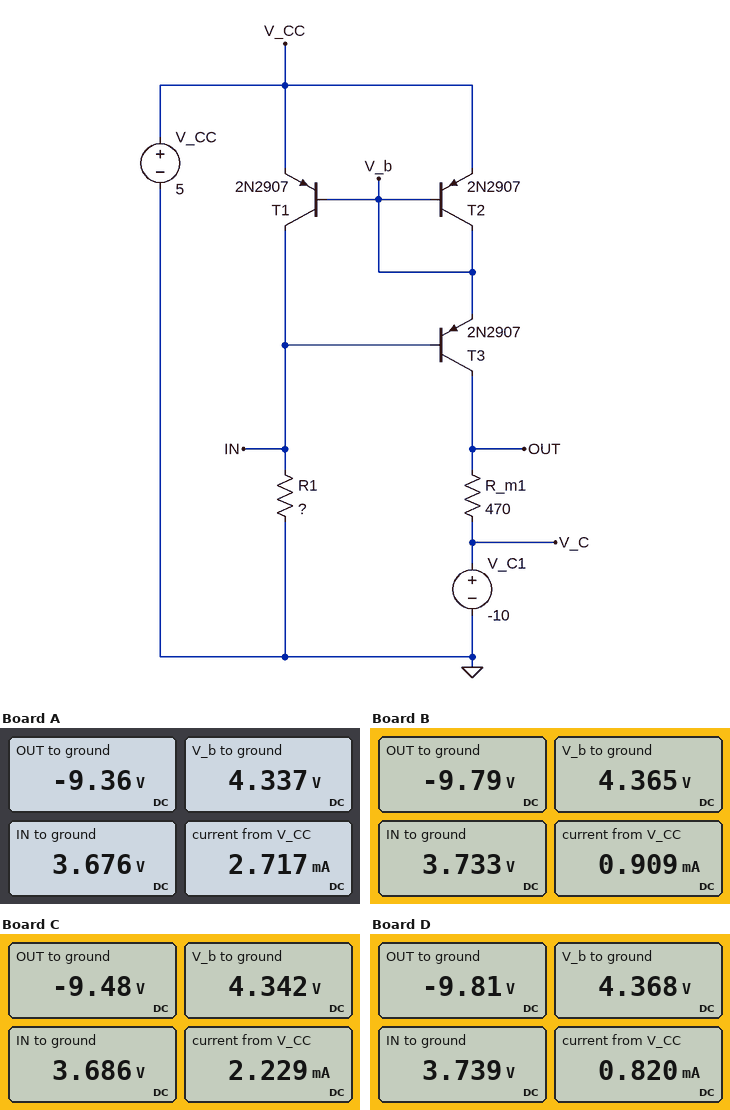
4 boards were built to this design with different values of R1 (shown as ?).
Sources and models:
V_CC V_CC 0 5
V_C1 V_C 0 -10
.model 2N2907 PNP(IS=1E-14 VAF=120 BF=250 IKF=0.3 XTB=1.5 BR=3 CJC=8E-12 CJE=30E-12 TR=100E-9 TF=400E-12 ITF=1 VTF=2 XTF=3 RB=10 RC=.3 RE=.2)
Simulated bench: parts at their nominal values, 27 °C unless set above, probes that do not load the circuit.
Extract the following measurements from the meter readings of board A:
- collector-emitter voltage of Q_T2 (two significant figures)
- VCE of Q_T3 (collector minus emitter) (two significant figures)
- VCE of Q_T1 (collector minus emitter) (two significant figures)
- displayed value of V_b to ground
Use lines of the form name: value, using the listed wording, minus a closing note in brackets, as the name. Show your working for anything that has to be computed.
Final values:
collector-emitter voltage of Q_T2: 4.337 V - 5 V = -660 mV
VCE of Q_T3 (collector minus emitter): -9.36 V - 4.337 V = -14 V
VCE of Q_T1 (collector minus emitter): 3.676 V - 5 V = -1.3 V
displayed value of V_b to ground: 4.337 V
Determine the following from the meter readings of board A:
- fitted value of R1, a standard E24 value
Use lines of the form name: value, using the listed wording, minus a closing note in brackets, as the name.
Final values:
fitted value of R1, a standard E24 value: 2.7 kΩ
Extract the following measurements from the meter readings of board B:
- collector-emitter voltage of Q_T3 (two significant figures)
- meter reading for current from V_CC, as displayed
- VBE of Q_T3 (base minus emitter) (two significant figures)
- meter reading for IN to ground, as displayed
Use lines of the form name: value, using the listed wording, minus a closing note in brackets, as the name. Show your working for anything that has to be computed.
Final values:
collector-emitter voltage of Q_T3: -9.79 V - 4.365 V = -14 V
meter reading for current from V_CC, as displayed: 0.909 mA
VBE of Q_T3 (base minus emitter): 3.733 V - 4.365 V = -630 mV
meter reading for IN to ground, as displayed: 3.733 V
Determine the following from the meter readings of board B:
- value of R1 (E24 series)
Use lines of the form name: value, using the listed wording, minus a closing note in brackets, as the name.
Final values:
value of R1: 8.2 kΩ
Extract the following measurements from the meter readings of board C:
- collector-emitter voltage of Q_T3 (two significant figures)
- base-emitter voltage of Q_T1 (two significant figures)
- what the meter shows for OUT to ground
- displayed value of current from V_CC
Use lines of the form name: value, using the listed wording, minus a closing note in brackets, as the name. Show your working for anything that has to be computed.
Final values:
collector-emitter voltage of Q_T3: -9.48 V - 4.342 V = -14 V
base-emitter voltage of Q_T1: 4.342 V - 5 V = -660 mV
what the meter shows for OUT to ground: -9.48 V
displayed value of current from V_CC: 2.229 mA
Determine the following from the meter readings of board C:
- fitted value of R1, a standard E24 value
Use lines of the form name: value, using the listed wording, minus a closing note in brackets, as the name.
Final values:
fitted value of R1, a standard E24 value: 3.3 kΩ
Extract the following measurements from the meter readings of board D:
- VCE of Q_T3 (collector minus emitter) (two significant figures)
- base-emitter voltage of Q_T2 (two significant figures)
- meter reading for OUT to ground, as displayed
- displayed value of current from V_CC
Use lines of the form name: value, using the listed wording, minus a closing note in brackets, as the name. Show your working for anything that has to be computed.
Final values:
VCE of Q_T3 (collector minus emitter): -9.81 V - 4.368 V = -14 V
base-emitter voltage of Q_T2: 4.368 V - 5 V = -630 mV
meter reading for OUT to ground, as displayed: -9.81 V
displayed value of current from V_CC: 0.820 mA
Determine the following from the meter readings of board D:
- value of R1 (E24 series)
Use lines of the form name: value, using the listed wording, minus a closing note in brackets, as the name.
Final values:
value of R1: 9.1 kΩ
